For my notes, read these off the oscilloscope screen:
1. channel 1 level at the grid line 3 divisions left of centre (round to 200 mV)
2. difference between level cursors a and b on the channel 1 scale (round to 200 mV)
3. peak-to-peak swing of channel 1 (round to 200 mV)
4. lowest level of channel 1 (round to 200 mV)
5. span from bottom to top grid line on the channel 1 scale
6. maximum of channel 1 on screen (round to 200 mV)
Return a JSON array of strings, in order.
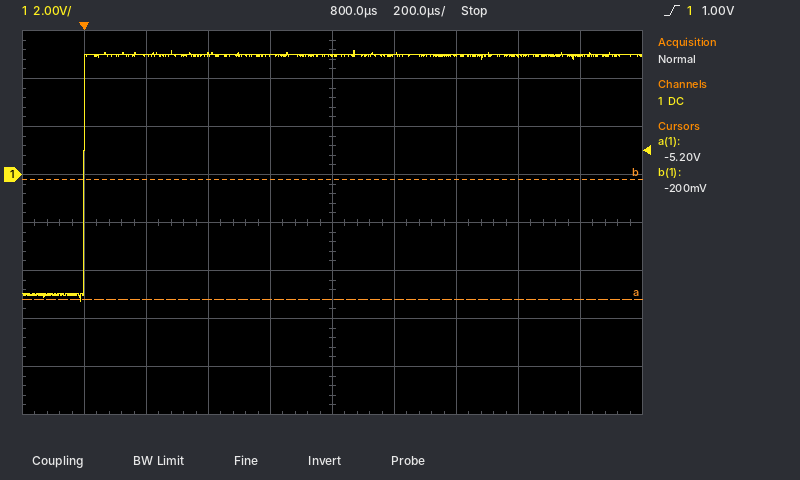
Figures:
["5.0 V", "5.0 V", "10.4 V", "-5.2 V", "16 V", "5.2 V"]
